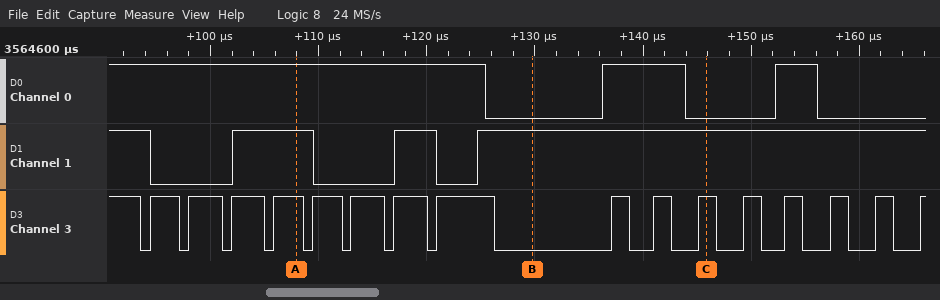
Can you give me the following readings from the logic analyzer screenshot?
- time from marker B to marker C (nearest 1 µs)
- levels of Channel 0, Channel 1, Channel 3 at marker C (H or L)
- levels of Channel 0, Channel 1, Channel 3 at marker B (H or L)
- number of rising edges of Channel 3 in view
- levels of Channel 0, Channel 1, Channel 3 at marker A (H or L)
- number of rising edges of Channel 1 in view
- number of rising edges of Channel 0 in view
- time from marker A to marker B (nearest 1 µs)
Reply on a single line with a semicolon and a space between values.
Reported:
16 µs; Channel 0=L, Channel 1=H, Channel 3=H; Channel 0=L, Channel 1=H, Channel 3=L; 16; Channel 0=H, Channel 1=H, Channel 3=H; 3; 2; 22 µs
